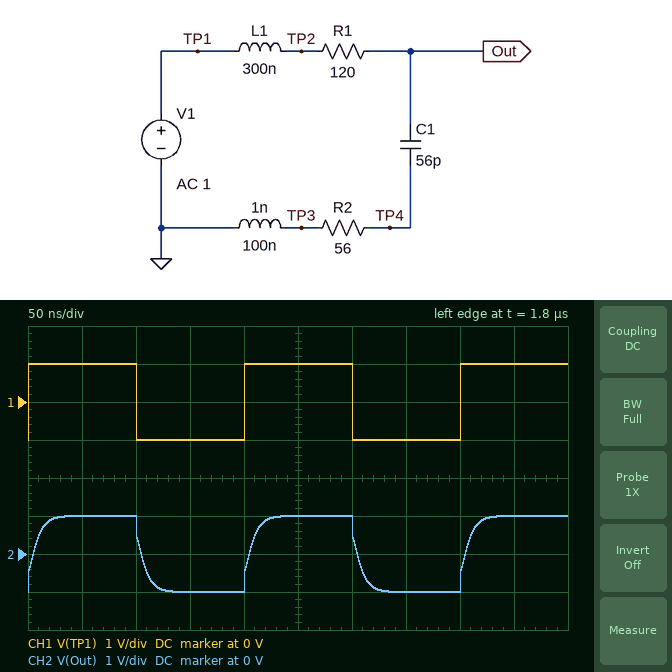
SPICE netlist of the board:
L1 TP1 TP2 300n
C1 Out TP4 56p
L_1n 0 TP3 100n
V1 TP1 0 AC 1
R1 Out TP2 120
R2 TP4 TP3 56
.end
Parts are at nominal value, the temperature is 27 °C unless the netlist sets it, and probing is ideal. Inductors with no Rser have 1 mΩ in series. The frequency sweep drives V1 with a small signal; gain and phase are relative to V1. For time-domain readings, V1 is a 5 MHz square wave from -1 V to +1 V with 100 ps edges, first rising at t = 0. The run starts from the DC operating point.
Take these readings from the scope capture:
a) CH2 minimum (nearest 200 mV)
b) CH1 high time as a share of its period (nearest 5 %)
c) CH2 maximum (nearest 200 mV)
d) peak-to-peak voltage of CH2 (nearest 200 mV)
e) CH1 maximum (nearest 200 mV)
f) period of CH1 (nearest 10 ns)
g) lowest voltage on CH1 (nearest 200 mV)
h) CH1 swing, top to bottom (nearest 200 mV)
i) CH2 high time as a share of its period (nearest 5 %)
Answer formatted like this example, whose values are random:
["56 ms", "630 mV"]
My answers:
["-1.0 V", "50 %", "1.0 V", "2.0 V", "1.0 V", "200 ns", "-1.0 V", "2.0 V", "50 %"]
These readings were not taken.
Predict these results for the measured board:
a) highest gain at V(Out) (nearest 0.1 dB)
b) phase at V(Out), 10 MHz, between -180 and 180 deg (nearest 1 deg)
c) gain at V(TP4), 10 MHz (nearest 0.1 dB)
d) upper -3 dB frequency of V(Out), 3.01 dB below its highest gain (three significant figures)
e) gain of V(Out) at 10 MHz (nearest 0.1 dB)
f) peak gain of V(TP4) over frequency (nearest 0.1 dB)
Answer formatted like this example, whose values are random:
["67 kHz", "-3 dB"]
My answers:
["0 dB", "-23 deg", "-14.9 dB", "20.2 MHz", "-0.9 dB", "-9.3 dB"]
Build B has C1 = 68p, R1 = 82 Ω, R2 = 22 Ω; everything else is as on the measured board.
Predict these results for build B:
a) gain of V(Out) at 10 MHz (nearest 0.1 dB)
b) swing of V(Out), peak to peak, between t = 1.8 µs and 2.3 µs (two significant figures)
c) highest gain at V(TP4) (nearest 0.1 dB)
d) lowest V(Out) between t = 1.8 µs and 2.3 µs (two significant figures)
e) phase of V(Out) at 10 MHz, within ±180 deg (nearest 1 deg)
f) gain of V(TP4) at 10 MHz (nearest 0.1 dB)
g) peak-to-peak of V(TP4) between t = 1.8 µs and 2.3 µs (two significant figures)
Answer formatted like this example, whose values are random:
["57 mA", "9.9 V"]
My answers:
["-0.2 dB", "2.2 V", "-10.5 dB", "-1.1 V", "-21 deg", "-20.2 dB", "1.0 V"]
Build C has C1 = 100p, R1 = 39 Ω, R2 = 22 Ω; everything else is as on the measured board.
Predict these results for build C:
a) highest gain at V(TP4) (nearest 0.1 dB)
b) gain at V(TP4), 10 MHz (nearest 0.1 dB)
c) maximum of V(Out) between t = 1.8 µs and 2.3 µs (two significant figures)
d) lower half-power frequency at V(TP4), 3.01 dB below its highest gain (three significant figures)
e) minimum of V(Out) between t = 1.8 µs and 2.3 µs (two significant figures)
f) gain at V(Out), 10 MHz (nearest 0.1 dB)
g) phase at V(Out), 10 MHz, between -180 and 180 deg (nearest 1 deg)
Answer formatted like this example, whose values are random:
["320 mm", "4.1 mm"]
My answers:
["-6.9 dB", "-16.2 dB", "1.3 V", "17.5 MHz", "-1.3 V", "0.4 dB", "-16 deg"]
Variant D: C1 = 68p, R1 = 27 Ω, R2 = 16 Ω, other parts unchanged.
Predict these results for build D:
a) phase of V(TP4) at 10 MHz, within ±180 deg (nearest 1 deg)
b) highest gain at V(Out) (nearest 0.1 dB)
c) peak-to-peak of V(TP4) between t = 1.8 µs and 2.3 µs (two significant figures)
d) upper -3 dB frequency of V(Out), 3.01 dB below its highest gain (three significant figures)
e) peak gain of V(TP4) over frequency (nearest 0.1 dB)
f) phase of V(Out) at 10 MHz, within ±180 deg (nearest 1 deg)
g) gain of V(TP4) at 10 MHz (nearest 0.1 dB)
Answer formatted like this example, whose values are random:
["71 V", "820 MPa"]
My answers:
["100 deg", "3.7 dB", "1.0 V", "34.1 MHz", "-4.6 dB", "-8 deg", "-21.9 dB"]
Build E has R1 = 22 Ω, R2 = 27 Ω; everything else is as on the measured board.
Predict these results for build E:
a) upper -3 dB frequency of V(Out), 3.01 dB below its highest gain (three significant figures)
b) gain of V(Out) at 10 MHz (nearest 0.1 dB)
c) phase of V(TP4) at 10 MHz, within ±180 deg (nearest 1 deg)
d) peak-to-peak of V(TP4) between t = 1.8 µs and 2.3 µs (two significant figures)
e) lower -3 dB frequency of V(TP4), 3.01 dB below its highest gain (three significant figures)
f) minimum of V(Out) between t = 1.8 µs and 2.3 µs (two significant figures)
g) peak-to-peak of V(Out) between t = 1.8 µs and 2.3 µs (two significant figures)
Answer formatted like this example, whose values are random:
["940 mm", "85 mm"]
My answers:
["38.0 MHz", "0.5 dB", "92 deg", "1.2 V", "26.5 MHz", "-1.6 V", "3.2 V"]
